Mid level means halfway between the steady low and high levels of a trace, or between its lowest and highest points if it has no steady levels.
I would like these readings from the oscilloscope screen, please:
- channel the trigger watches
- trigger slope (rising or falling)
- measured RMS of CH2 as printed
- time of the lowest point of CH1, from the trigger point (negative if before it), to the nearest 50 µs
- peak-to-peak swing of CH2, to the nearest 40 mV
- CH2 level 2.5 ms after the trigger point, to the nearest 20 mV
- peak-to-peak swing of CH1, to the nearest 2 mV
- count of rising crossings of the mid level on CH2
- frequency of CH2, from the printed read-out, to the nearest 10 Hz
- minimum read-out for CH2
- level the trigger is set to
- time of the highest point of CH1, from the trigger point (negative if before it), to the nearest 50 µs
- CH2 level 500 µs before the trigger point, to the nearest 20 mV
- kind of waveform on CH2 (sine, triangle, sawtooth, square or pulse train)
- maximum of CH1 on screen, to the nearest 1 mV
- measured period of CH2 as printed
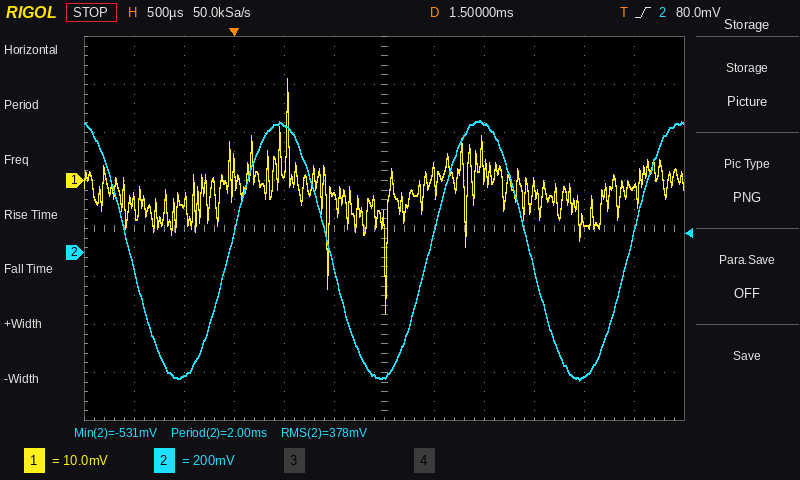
CH2
rising
378 mV
+1.50 ms
1.08 V
540 mV
48 mV
3
500 Hz
-531 mV
80.0 mV
+550 µs
-520 mV
sine
21 mV
2.00 ms
